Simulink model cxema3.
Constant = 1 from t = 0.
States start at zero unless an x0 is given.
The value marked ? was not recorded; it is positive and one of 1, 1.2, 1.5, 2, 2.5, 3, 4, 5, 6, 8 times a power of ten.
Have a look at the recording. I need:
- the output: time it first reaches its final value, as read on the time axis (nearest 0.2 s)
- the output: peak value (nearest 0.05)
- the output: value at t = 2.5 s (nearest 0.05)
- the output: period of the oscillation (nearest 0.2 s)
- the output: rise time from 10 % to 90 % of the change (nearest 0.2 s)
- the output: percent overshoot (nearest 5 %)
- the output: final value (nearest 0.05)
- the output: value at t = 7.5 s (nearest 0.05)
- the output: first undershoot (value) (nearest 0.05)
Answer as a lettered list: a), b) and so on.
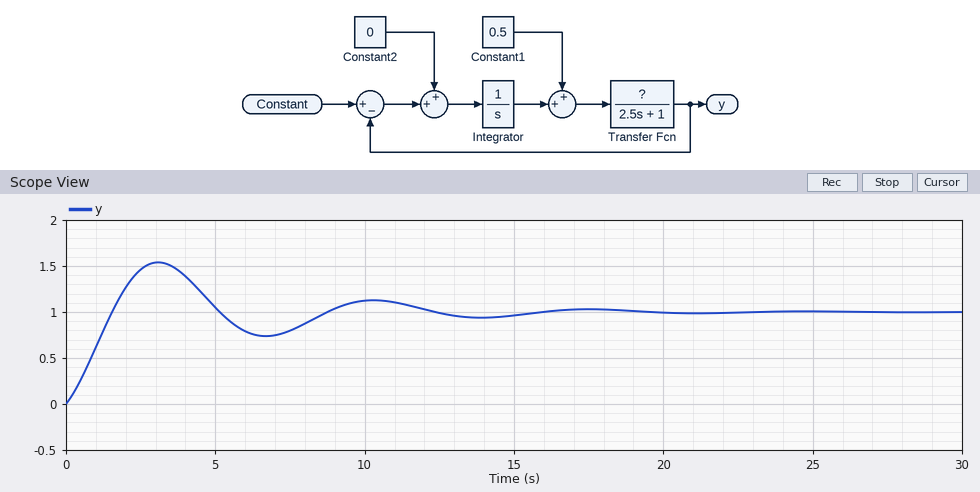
a) 1.6 s
b) 1.55
c) 1.45
d) 7.2 s
e) 1.2 s
f) 55 %
g) 1.00
h) 0.80
i) 0.75
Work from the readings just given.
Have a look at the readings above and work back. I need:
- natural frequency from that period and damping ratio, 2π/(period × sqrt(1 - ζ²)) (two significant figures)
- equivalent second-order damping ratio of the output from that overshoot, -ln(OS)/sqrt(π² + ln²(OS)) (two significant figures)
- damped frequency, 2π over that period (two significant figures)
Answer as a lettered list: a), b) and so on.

a) 0.89 rad/s
b) 0.19
c) 0.87 rad/s
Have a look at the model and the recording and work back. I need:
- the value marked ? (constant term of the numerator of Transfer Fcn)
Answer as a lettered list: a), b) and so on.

a) 2
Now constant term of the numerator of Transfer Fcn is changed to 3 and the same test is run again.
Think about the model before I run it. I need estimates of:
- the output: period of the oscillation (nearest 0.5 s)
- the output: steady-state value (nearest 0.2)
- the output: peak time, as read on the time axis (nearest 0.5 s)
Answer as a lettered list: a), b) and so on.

a) 6.0 s
b) 1.0
c) 2.5 s
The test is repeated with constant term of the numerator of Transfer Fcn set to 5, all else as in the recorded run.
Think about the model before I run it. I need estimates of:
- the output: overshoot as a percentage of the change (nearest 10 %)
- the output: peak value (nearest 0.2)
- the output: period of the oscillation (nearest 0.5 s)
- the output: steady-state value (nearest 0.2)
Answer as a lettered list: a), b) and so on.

a) 80 %
b) 1.8
c) 4.5 s
d) 1.0
